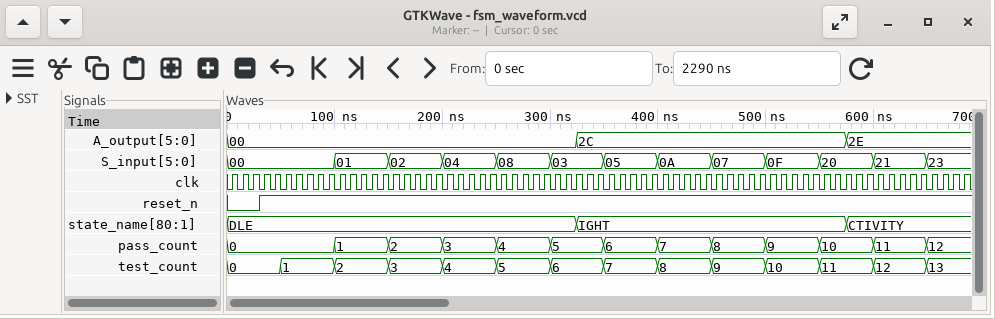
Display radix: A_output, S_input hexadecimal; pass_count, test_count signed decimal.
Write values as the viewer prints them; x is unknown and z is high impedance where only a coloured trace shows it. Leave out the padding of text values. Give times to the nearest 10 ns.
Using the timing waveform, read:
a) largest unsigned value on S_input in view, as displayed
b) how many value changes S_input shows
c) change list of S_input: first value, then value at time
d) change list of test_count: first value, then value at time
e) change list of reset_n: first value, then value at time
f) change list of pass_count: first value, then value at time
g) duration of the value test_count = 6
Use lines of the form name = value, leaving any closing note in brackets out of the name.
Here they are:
largest unsigned value on S_input in view, as displayed = 23
how many value changes S_input shows = 12
change list of S_input: first value, then value at time = 00, 01 at 100 ns, 02 at 150 ns, 04 at 200 ns, 08 at 250 ns, 03 at 300 ns, 05 at 350 ns, 0A at 400 ns, 07 at 450 ns, 0F at 500 ns, 20 at 550 ns, 21 at 600 ns, 23 at 650 ns
change list of test_count: first value, then value at time = 0, 1 at 50 ns, 2 at 100 ns, 3 at 150 ns, 4 at 200 ns, 5 at 250 ns, 6 at 300 ns, 7 at 350 ns, 8 at 400 ns, 9 at 450 ns, 10 at 500 ns, 11 at 550 ns, 12 at 600 ns, 13 at 650 ns
change list of reset_n: first value, then value at time = 0, 1 at 30 ns
change list of pass_count: first value, then value at time = 0, 1 at 100 ns, 2 at 150 ns, 3 at 200 ns, 4 at 250 ns, 5 at 300 ns, 6 at 350 ns, 7 at 400 ns, 8 at 450 ns, 9 at 500 ns, 10 at 550 ns, 11 at 600 ns, 12 at 650 ns
duration of the value test_count = 6 = 50 ns
